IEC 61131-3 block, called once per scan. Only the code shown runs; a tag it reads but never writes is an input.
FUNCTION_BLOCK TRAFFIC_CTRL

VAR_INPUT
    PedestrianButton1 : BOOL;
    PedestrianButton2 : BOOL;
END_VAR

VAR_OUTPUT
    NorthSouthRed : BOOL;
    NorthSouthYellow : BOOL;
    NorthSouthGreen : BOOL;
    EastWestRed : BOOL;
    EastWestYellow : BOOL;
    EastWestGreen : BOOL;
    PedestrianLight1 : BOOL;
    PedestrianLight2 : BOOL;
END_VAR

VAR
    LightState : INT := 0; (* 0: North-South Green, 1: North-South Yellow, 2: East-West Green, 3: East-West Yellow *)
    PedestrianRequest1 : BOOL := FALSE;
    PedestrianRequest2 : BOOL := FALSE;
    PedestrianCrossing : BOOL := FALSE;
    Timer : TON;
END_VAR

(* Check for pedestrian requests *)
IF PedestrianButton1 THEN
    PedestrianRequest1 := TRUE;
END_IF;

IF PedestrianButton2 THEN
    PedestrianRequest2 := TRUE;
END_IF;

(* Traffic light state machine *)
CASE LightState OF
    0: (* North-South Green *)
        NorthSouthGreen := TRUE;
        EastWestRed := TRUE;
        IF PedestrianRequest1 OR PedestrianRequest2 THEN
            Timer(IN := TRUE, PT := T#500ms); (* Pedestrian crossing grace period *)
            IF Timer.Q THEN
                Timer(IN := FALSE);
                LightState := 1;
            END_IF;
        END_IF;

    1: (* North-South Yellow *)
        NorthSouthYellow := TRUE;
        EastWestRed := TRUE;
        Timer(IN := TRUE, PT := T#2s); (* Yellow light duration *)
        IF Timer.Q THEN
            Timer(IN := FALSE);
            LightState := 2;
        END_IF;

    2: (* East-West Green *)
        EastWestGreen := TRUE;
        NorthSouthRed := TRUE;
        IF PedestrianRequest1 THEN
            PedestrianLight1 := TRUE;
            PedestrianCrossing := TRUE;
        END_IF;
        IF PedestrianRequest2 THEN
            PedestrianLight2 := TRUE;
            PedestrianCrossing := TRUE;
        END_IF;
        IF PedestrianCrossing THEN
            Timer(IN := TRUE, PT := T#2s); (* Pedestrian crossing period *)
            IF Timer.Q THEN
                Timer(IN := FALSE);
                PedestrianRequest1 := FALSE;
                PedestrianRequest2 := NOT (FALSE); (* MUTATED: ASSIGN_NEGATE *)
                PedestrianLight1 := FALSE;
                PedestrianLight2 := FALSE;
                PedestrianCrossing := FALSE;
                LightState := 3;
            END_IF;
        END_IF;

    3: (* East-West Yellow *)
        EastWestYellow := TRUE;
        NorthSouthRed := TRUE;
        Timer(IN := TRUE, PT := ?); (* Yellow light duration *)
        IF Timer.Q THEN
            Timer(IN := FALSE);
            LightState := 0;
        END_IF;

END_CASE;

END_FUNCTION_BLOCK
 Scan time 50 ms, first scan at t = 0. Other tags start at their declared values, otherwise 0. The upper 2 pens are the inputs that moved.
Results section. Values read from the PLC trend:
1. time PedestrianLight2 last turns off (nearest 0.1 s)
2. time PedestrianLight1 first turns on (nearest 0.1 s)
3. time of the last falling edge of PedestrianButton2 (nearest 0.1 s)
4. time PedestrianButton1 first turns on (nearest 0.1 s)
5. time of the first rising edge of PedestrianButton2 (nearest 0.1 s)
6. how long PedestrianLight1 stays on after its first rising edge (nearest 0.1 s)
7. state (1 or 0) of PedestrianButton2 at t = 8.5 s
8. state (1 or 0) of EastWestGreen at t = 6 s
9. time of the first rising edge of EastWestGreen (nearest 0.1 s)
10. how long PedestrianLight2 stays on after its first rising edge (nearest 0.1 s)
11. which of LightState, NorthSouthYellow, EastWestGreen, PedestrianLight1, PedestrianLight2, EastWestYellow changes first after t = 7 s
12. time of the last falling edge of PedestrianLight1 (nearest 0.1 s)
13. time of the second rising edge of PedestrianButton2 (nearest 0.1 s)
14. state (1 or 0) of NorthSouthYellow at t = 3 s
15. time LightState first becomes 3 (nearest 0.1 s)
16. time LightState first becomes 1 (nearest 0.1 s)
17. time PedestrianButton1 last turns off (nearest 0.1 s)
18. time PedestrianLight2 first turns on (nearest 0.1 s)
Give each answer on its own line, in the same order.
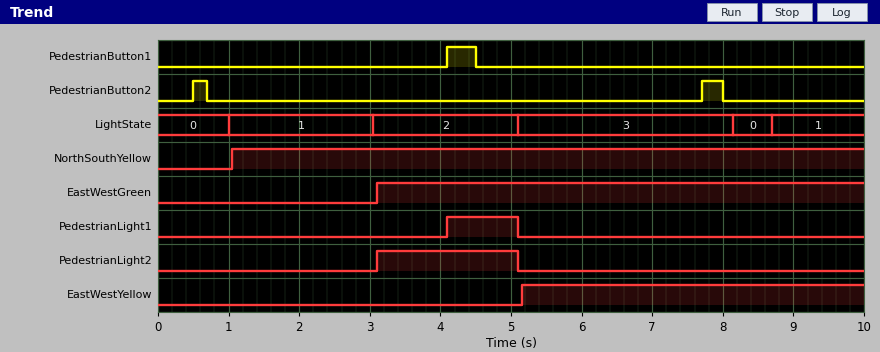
5.1 s
4.1 s
8.0 s
4.1 s
0.5 s
1.0 s
0
1
3.1 s
2.0 s
LightState
5.1 s
7.7 s
1
5.1 s
1.0 s
4.5 s
3.1 s
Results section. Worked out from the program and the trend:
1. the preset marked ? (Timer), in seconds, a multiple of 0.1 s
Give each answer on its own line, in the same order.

3.0 s
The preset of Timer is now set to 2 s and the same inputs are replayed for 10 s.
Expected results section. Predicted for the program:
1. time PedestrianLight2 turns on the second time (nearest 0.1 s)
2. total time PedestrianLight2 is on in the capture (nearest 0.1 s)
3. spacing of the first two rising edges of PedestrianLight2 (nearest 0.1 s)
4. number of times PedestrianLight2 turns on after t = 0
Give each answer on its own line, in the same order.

9.8 s
2.2 s
6.7 s
2
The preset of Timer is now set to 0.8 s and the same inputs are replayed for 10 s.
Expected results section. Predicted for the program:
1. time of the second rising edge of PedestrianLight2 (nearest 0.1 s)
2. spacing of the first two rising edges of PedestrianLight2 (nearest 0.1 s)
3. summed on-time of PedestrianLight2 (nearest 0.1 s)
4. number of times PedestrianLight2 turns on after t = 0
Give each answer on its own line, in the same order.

8.6 s
5.5 s
3.4 s
2
